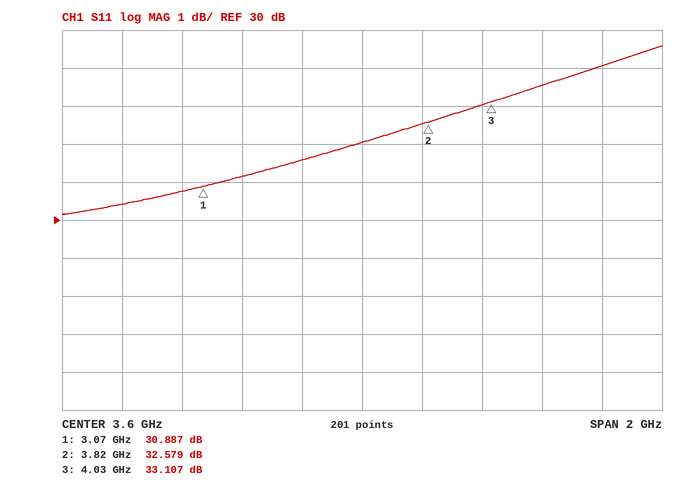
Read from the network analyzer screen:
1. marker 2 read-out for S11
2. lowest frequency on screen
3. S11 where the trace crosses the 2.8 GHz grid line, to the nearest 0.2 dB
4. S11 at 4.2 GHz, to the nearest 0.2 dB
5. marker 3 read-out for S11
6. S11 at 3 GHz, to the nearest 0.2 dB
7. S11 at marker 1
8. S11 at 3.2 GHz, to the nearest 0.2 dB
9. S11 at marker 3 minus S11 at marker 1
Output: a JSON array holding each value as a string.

["32.579 dB", "2.6 GHz", "30.4 dB", "33.6 dB", "33.107 dB", "30.8 dB", "30.887 dB", "31.2 dB", "2.220 dB"]
